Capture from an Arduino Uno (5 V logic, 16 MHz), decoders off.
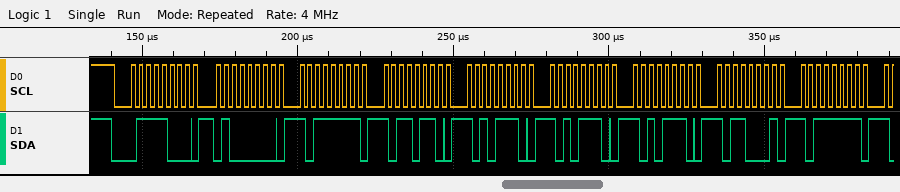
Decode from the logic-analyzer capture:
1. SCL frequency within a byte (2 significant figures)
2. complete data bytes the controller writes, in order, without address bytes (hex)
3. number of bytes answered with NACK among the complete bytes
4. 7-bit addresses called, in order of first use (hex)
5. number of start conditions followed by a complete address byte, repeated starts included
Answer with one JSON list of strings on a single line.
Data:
["400 kHz", "40 BF B6 AE AE AE B1 BF", "0", "0x3C", "1"]
